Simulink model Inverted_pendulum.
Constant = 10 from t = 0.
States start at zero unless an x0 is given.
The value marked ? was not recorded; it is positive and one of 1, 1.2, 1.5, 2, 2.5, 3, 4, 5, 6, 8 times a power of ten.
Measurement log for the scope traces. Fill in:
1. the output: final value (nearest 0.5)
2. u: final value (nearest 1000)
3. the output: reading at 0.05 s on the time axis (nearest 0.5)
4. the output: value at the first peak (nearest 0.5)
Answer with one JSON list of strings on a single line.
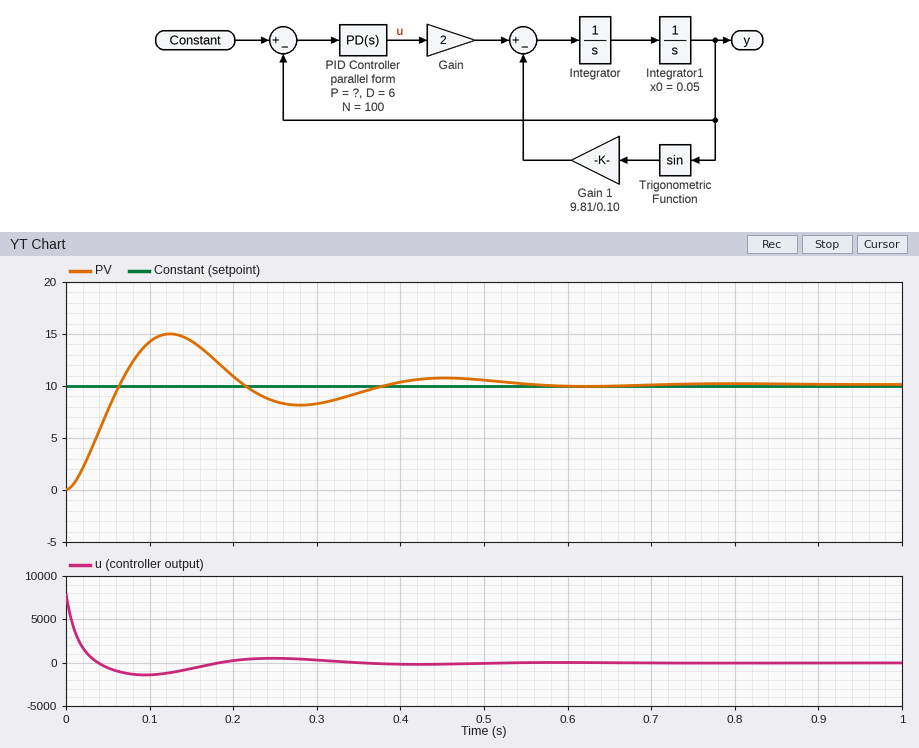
["10.0", "0", "7.5", "15.0"]
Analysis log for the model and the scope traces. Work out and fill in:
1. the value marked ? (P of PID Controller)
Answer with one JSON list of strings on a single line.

["200"]
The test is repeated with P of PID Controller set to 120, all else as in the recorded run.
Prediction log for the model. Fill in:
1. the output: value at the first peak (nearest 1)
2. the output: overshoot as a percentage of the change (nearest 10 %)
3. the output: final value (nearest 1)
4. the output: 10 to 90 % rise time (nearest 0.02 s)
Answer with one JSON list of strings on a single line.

["14", "40 %", "10", "0.06 s"]
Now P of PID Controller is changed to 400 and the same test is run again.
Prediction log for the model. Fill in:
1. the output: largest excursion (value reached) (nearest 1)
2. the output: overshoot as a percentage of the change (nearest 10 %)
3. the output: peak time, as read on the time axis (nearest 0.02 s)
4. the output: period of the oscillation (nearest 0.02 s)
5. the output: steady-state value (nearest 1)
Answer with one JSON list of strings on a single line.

["16", "60 %", "0.10 s", "0.22 s", "10"]
